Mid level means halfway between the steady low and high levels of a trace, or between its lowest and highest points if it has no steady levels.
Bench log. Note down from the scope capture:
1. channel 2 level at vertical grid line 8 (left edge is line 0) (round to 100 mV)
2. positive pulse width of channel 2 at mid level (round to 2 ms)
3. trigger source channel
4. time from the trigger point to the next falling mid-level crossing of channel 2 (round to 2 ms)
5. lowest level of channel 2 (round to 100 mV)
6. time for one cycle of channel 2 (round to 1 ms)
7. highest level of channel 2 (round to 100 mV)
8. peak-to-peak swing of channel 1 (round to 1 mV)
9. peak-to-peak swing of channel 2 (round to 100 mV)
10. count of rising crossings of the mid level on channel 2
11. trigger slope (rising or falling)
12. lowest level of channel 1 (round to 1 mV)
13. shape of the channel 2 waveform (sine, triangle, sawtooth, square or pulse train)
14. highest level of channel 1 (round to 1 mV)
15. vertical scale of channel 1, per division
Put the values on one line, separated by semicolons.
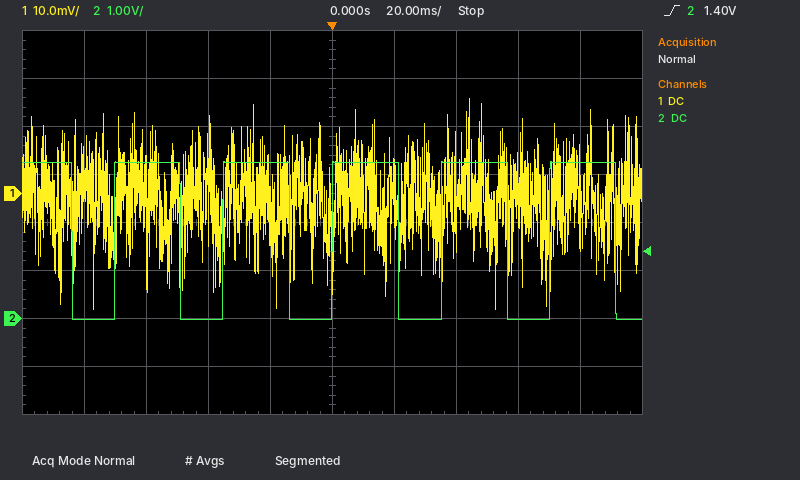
0.0 V; 22 ms; channel 2; 22 ms; 0.0 V; 35 ms; 3.3 V; 44 mV; 3.3 V; 5; rising; -24 mV; pulse train; 20 mV; 10 mV
